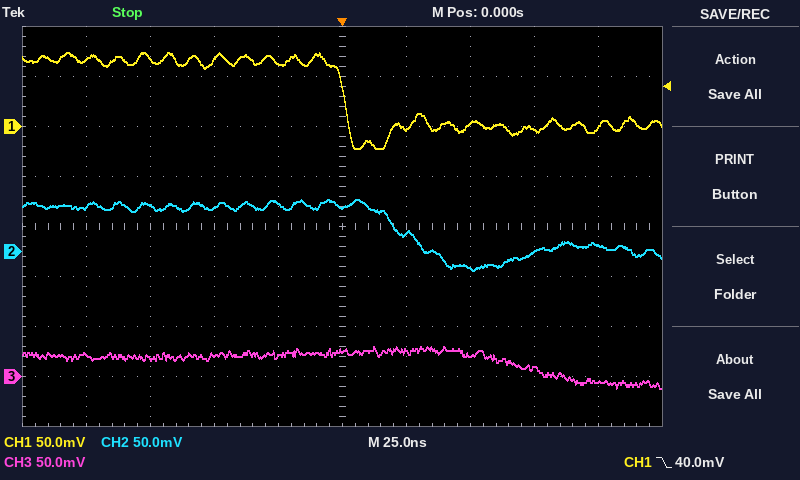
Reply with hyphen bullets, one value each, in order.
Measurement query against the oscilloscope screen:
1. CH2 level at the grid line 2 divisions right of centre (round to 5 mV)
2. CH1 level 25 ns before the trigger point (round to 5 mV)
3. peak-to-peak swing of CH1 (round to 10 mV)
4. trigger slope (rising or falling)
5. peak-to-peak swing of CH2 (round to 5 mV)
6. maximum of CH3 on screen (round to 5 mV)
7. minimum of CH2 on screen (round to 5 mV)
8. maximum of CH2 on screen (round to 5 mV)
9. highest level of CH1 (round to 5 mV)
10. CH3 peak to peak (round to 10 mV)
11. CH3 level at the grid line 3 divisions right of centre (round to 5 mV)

- -15 mV
- 65 mV
- 100 mV
- falling
- 70 mV
- 30 mV
- -20 mV
- 50 mV
- 75 mV
- 40 mV
- 10 mV
